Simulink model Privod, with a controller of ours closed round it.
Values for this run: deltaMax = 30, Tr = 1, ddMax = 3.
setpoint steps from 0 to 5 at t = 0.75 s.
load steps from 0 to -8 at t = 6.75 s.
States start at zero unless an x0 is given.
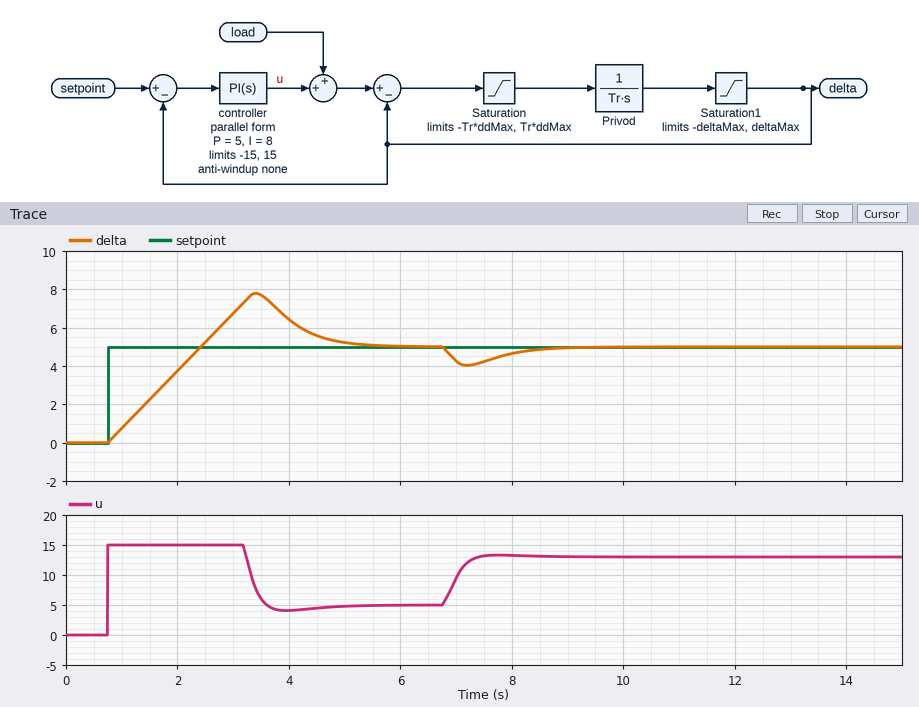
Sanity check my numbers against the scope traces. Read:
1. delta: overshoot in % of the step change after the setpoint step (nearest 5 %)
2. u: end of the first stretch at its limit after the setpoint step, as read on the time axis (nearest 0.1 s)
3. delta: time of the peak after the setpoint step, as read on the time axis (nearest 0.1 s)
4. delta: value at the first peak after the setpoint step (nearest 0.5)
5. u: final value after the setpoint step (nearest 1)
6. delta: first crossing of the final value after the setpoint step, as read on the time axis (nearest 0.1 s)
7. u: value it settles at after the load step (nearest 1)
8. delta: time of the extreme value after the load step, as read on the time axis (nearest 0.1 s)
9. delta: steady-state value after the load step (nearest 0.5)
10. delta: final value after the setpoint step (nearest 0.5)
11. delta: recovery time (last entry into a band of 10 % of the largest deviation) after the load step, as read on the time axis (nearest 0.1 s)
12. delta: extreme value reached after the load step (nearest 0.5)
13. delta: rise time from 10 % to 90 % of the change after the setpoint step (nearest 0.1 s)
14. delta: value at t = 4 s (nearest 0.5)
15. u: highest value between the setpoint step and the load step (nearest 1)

55 %
3.2 s
3.4 s
8.0
5
2.4 s
13
7.2 s
5.0
5.0
8.7 s
4.0
1.3 s
6.5
15
